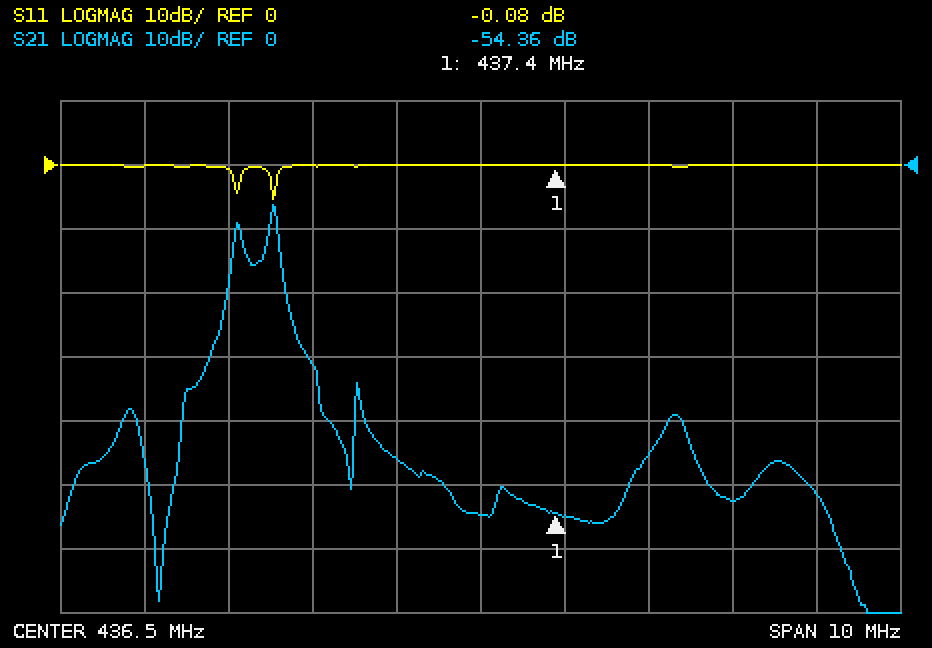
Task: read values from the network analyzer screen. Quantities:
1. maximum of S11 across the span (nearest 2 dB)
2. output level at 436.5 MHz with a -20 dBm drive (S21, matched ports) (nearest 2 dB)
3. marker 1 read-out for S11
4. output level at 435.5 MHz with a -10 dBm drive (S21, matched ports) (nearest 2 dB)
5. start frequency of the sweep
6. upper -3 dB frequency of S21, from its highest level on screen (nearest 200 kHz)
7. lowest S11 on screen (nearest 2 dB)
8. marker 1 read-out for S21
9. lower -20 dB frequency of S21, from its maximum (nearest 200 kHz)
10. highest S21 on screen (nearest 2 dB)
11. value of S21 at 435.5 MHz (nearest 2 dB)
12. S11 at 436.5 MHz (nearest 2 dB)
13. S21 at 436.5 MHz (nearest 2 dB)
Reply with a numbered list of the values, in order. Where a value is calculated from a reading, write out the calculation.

1. 0 dB
2. -20 dBm + (-54 dB) = -74 dBm
3. -0.08 dB
4. -10 dBm + (-46 dB) = -56 dBm
5. 431.5 MHz
6. 434.0 MHz
7. -6 dB
8. -54.36 dB
9. 433.4 MHz
10. -6 dB
11. -46 dB
12. 0 dB
13. -54 dB
